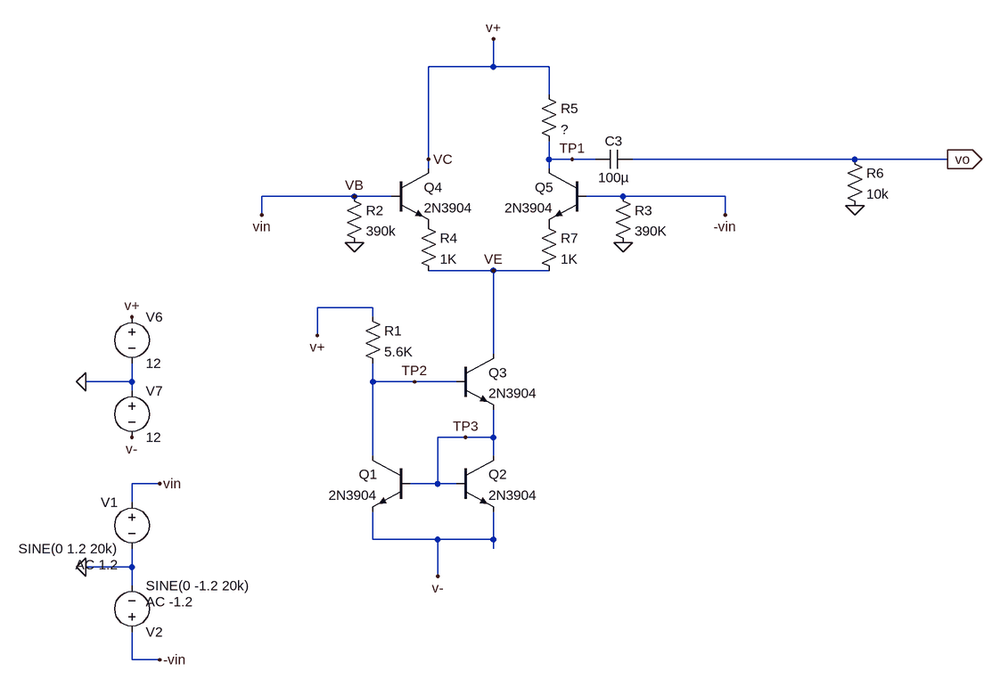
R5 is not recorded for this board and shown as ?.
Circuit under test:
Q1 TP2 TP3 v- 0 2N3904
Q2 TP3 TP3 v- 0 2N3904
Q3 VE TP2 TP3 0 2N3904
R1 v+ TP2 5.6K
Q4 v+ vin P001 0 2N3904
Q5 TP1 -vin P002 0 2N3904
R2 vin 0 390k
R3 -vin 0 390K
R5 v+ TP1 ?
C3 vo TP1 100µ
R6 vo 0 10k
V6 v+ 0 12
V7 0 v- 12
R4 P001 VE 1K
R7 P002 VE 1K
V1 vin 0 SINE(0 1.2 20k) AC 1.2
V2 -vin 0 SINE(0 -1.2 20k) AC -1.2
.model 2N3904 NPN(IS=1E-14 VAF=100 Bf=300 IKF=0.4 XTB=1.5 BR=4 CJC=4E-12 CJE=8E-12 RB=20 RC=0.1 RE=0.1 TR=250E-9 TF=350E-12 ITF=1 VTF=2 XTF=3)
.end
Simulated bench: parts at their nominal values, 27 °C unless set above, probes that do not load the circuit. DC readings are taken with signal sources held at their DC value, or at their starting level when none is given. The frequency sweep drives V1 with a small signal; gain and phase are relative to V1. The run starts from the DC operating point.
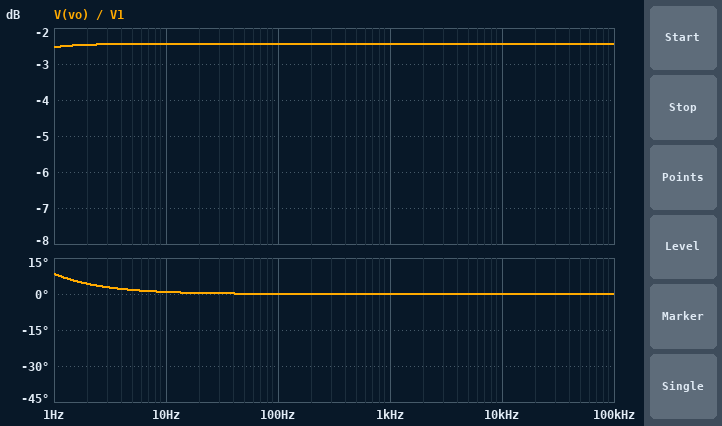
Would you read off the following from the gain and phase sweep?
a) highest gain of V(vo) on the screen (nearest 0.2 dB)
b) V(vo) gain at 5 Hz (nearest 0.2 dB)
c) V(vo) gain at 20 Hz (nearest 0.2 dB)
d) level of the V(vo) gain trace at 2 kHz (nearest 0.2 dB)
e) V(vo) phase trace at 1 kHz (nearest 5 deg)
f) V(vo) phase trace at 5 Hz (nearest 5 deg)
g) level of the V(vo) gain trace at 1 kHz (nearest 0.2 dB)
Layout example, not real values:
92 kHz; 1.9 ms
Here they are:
-2.4 dB; -2.4 dB; -2.4 dB; -2.4 dB; 0 deg; 0 deg; -2.4 dB
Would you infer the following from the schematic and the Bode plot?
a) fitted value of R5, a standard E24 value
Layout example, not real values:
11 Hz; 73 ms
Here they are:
750 Ω
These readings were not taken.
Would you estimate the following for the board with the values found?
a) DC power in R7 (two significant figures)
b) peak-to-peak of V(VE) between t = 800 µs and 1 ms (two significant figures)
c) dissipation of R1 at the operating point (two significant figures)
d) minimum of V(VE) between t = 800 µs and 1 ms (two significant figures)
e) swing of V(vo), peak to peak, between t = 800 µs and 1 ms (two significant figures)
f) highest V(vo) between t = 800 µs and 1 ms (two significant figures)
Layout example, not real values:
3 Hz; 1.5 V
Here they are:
4.0 mW; 5.6 mV; 91 mW; -2.7 V; 1.6 V; 820 mV
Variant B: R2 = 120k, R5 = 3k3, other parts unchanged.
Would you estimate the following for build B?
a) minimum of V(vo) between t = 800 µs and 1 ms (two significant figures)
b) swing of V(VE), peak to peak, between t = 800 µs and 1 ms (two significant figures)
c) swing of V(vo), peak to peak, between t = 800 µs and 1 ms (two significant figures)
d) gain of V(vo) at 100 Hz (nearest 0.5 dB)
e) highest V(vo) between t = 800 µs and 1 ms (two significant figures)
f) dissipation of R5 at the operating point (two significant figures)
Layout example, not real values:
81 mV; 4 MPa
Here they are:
-2.9 V; 5.9 mV; 5.8 V; 8.5 dB; 2.9 V; 13 mW
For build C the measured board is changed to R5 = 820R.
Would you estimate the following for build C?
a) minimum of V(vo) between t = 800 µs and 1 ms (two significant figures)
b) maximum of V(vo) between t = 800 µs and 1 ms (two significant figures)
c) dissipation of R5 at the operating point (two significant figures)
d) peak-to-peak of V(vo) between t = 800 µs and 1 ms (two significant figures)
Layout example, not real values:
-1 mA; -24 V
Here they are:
-890 mV; 890 mV; 3.3 mW; 1.8 V
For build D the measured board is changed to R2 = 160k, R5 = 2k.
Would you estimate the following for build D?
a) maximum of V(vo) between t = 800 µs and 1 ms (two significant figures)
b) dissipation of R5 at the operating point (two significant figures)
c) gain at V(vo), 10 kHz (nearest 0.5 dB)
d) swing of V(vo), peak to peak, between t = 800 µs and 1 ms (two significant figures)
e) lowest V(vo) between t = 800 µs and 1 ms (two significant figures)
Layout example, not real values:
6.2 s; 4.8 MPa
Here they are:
2.0 V; 8.0 mW; 5.0 dB; 3.9 V; -2.0 V
